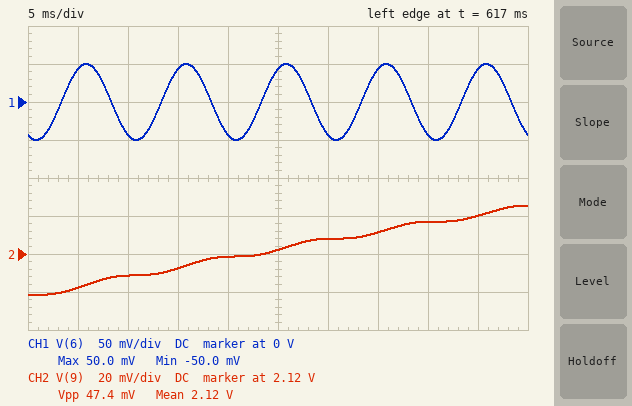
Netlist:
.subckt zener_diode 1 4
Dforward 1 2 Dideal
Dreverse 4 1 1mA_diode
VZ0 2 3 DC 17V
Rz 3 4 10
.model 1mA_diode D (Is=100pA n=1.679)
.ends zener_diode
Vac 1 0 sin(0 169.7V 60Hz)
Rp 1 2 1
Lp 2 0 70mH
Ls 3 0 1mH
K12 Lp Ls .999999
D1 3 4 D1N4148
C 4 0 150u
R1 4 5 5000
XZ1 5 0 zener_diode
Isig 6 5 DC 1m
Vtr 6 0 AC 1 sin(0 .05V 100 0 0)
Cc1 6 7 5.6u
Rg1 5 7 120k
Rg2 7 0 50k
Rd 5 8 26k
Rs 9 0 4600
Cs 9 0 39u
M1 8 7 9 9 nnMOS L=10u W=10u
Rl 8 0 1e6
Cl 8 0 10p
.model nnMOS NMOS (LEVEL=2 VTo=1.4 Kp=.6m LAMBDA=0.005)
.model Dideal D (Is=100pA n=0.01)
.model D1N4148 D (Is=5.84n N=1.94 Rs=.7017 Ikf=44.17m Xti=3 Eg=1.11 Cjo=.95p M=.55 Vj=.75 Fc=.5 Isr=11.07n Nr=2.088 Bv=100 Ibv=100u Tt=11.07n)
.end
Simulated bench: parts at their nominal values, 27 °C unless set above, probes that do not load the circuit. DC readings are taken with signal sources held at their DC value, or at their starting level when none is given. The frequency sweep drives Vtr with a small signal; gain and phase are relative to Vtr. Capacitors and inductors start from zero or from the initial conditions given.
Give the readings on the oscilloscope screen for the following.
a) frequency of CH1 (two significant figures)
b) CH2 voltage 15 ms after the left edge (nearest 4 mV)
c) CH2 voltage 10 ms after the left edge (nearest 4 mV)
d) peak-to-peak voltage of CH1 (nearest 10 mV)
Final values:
100 Hz
2.112 V
2.108 V
100 mV
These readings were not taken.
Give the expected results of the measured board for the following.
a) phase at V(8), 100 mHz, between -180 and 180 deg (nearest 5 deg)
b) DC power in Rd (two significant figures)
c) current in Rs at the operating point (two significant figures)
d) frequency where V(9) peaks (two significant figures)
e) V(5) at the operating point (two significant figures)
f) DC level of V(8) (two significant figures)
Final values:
-90 deg
6.7 mW
500 µA
1.8 Hz
17 V
3.8 V
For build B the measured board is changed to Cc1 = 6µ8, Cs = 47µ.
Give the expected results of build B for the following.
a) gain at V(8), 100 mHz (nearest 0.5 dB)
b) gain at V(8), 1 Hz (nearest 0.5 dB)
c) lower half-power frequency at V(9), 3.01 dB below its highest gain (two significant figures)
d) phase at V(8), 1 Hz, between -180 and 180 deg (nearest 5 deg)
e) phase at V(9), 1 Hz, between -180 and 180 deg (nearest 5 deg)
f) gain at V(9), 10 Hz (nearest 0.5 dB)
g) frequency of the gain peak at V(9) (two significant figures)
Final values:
-4.0 dB
15.0 dB
490 mHz
-110 deg
15 deg
-12.5 dB
1.5 Hz
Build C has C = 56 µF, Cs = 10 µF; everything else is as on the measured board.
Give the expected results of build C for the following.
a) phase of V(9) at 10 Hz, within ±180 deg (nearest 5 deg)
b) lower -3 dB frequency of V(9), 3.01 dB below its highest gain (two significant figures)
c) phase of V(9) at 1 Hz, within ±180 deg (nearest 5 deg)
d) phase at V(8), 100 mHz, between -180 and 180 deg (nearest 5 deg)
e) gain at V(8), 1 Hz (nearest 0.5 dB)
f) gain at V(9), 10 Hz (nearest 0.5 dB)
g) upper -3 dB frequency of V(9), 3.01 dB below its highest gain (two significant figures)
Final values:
-30 deg
730 mHz
35 deg
-95 deg
10.5 dB
-4.0 dB
17 Hz
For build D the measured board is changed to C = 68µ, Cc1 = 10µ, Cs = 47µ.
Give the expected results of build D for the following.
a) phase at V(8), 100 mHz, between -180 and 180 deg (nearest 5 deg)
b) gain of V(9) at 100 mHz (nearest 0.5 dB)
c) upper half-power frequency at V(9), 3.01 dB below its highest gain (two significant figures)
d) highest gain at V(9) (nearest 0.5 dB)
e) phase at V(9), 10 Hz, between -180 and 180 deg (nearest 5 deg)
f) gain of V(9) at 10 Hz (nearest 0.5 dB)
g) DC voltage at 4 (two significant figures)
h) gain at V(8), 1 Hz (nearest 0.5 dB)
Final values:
-95 deg
-15.5 dB
4.0 Hz
-3.5 dB
-70 deg
-12.5 dB
17 V
16.0 dB
